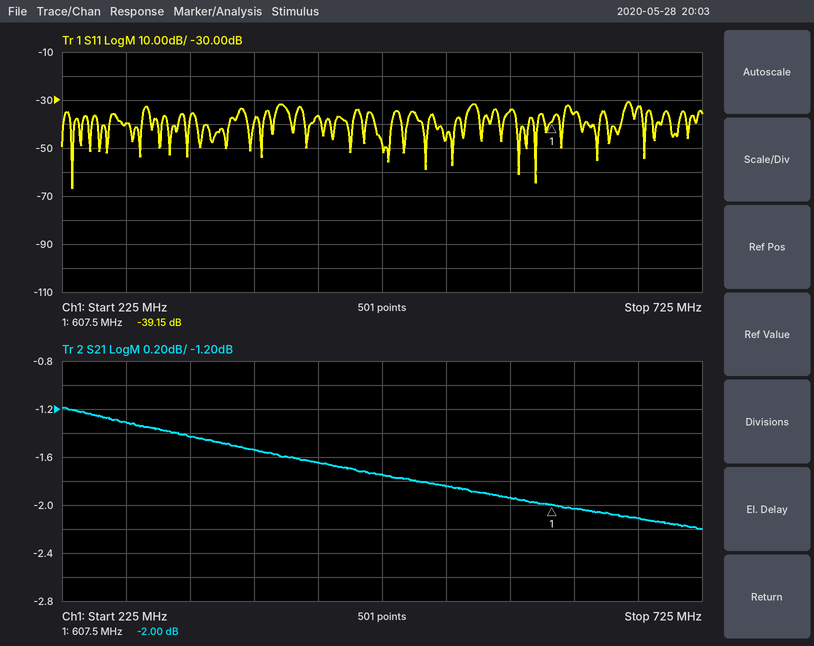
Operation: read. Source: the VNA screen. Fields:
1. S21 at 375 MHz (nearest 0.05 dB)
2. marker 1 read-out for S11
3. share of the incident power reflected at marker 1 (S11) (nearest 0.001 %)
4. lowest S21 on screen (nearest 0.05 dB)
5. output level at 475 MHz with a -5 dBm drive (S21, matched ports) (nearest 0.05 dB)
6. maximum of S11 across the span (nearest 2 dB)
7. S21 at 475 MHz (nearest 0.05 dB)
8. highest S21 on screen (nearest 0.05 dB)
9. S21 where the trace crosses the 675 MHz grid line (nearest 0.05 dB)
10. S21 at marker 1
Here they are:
-1.55 dB
-39.15 dB
0.012 %
-2.20 dB
-6.75 dBm
-30 dB
-1.75 dB
-1.20 dB
-2.10 dB
-2.00 dB
